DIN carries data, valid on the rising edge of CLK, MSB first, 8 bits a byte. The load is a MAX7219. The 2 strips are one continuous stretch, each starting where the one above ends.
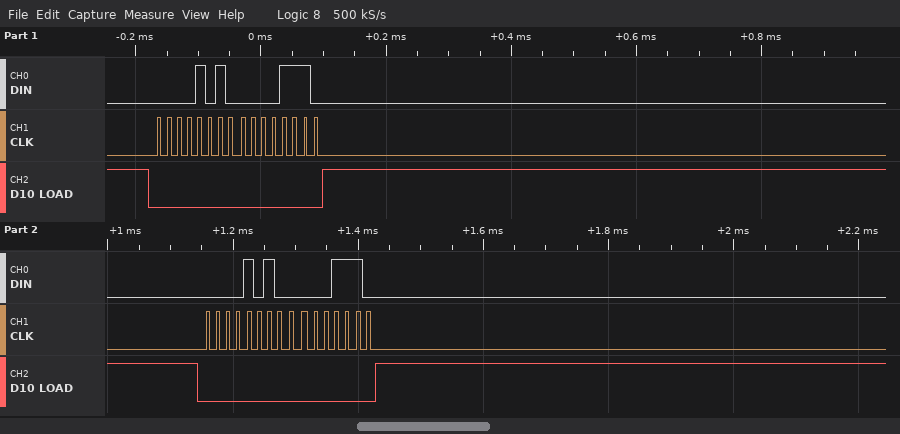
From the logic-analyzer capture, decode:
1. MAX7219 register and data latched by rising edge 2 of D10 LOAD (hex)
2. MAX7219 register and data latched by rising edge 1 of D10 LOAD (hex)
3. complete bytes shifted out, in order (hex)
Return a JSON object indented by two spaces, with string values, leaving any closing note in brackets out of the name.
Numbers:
{
  "MAX7219 register and data latched by rising edge 2 of D10 LOAD": "register 0xA, data 0x0E",
  "MAX7219 register and data latched by rising edge 1 of D10 LOAD": "register 0xA, data 0x0E",
  "complete bytes shifted out, in order": "0x0A 0x0E 0x0A 0x0E"
}
